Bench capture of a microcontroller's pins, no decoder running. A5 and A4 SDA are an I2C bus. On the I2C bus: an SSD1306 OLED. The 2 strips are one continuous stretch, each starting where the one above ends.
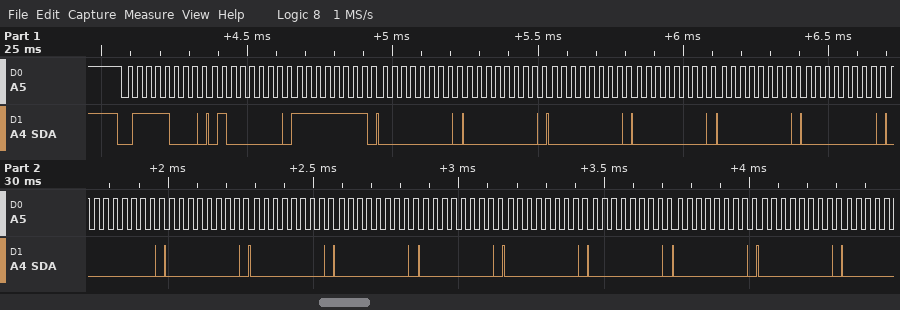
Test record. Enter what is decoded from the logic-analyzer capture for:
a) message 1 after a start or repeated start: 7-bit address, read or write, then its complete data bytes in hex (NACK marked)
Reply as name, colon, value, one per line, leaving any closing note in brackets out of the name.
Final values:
message 1 after a start or repeated start: 7-bit address, read or write, then its complete data bytes in hex: 0x3C write: 40 FF 00 00 00 00 00 00 00 00 00 00 00 00 00 00 00
